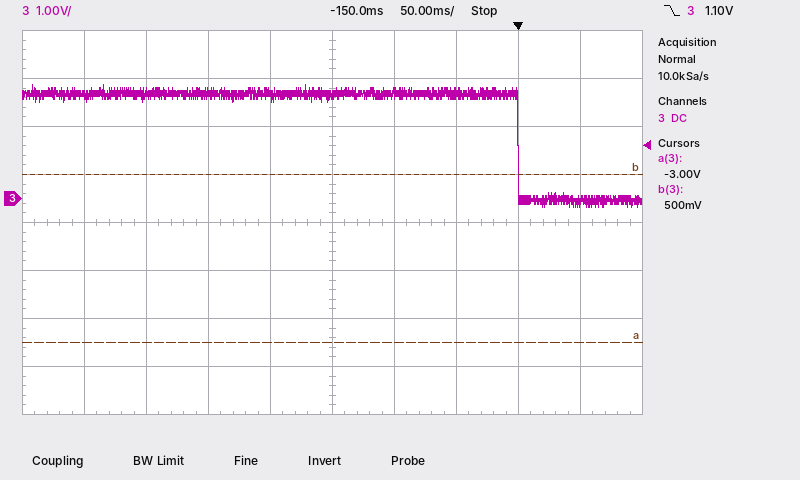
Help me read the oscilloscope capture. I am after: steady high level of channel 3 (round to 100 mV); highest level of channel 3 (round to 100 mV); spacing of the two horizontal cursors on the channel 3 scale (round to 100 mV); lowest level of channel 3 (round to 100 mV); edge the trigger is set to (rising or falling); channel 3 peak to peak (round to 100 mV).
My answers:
2.2 V
2.4 V
3.5 V
-200 mV
falling
2.6 V
